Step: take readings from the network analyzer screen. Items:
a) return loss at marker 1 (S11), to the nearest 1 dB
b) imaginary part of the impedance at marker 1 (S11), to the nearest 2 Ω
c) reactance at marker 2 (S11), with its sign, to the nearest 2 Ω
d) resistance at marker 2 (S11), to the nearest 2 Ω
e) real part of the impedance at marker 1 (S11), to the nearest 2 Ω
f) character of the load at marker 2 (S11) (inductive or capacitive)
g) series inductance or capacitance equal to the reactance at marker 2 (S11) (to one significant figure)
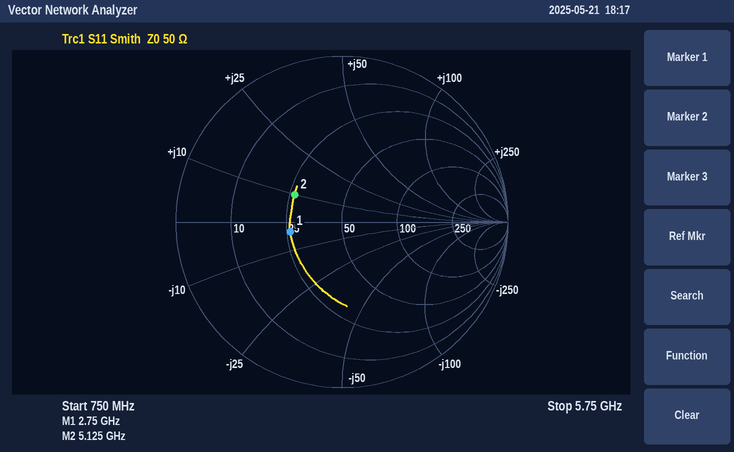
10 dB
-4 Ω
+10 Ω
26 Ω
26 Ω
inductive
300 pH
